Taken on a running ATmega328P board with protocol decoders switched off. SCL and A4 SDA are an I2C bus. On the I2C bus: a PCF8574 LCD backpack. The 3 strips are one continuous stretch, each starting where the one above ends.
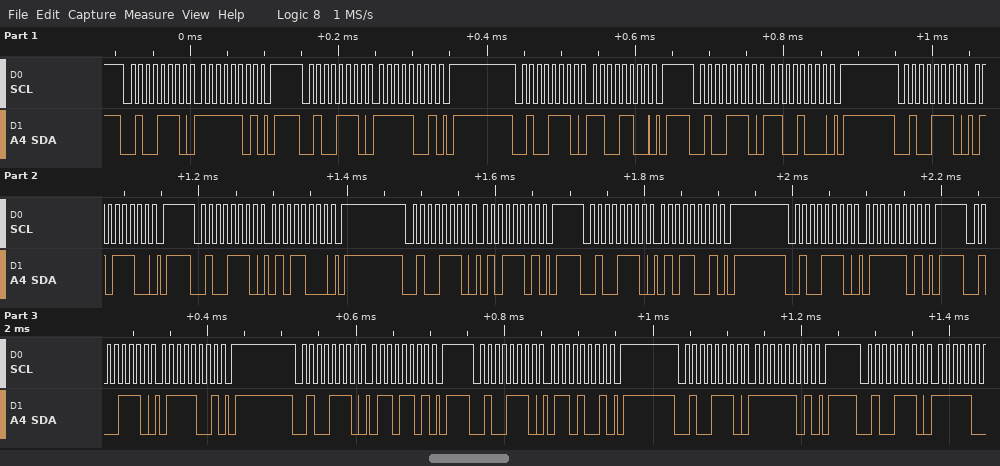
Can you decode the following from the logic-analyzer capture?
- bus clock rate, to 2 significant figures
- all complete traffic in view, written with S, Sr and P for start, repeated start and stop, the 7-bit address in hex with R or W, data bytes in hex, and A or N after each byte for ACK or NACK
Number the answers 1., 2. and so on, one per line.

1. 100 kHz
2. S 27W A FD A P S 27W A F9 A P S 27W A CC A P S 27W A C8 A P S 27W A 5C A P S 27W A 58 A P S 27W A 5D A P S 27W A 59 A P S 27W A 7D A P S 27W A 79 A P S 27W A 6D A P S 27W A 69 A P S 27W A FD A P S 27W A
